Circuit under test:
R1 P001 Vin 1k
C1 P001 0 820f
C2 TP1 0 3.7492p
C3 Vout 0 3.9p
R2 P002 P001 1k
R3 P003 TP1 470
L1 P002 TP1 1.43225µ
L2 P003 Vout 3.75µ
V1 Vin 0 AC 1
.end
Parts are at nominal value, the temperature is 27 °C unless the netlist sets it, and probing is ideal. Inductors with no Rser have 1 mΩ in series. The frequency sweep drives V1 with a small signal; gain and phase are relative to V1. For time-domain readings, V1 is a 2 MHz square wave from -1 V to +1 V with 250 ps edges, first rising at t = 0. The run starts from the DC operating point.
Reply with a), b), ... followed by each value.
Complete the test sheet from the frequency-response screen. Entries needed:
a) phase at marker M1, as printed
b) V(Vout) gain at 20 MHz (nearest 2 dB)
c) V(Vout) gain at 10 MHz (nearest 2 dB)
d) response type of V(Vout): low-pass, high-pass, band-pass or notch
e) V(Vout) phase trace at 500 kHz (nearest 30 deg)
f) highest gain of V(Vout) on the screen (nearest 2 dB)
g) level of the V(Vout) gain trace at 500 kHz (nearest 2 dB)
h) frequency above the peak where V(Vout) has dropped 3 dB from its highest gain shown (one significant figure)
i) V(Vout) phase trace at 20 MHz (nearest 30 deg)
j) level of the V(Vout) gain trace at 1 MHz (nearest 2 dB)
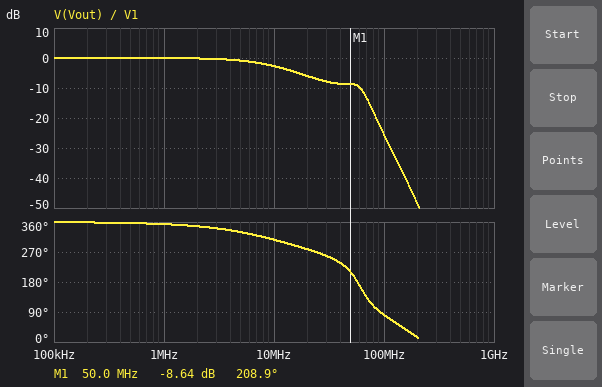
a) 208.9 deg
b) -6 dB
c) -2 dB
d) low-pass
e) 360 deg
f) 0 dB
g) 0 dB
h) 10 MHz
i) 270 deg
j) 0 dB
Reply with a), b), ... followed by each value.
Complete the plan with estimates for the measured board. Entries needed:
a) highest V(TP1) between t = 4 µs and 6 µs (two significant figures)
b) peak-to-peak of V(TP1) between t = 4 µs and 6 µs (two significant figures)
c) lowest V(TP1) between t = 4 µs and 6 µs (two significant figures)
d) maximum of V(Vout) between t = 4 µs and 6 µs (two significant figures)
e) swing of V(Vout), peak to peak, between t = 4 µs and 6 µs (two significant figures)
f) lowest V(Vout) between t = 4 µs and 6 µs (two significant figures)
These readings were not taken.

a) 1.0 V
b) 2.0 V
c) -1.0 V
d) 1.0 V
e) 2.0 V
f) -1.0 V
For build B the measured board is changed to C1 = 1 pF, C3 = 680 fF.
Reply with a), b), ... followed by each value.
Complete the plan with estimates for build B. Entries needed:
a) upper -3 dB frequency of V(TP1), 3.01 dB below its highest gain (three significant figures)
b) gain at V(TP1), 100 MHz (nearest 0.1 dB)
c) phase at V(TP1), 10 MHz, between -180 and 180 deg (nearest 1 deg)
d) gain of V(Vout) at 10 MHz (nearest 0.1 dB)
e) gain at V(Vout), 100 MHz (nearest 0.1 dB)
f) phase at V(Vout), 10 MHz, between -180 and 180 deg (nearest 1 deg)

a) 18.1 MHz
b) -17.1 dB
c) -33 deg
d) -1.1 dB
e) -3.2 dB
f) -34 deg
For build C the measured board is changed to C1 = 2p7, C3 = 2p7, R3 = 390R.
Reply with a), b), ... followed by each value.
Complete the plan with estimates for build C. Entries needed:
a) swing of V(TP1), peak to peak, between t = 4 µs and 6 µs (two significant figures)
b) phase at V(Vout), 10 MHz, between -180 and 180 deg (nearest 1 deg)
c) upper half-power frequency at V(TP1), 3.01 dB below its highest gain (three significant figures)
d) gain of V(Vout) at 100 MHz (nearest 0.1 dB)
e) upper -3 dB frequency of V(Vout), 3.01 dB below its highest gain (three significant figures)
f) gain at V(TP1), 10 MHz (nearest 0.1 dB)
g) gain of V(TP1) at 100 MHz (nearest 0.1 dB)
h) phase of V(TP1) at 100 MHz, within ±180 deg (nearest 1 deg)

a) 2.0 V
b) -51 deg
c) 11.0 MHz
d) -23.1 dB
e) 12.2 MHz
f) -2.6 dB
g) -13.3 dB
h) -142 deg
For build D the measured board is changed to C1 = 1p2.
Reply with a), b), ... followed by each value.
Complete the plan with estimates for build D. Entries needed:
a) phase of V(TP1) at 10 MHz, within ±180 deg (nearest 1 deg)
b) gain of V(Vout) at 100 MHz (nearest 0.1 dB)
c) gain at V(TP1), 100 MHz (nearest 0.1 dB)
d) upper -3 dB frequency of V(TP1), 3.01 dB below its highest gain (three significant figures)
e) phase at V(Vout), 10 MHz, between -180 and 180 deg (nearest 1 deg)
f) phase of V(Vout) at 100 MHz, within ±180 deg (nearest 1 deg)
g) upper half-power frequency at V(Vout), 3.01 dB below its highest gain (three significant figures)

a) -47 deg
b) -25.7 dB
c) -11.9 dB
d) 9.61 MHz
e) -54 deg
f) 74 deg
g) 10.7 MHz
